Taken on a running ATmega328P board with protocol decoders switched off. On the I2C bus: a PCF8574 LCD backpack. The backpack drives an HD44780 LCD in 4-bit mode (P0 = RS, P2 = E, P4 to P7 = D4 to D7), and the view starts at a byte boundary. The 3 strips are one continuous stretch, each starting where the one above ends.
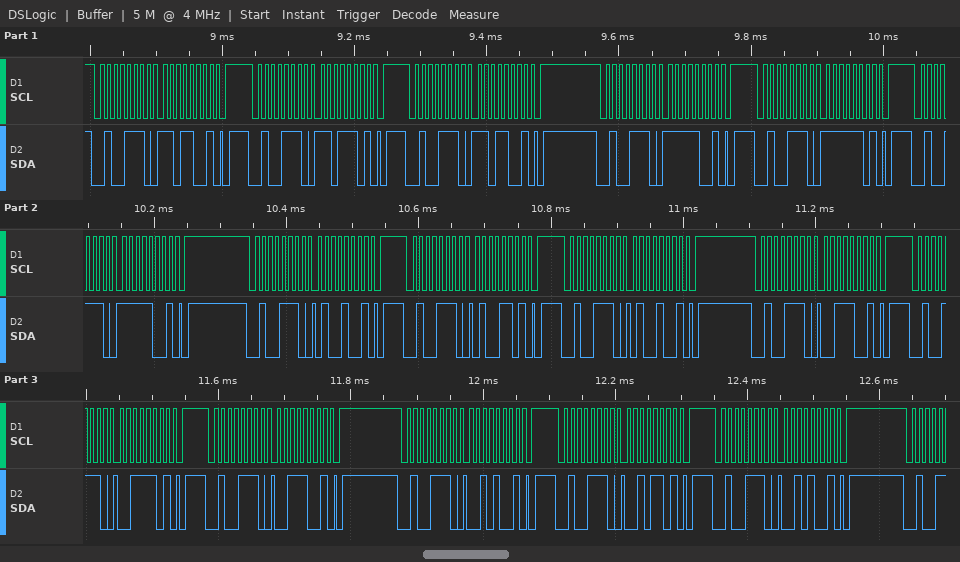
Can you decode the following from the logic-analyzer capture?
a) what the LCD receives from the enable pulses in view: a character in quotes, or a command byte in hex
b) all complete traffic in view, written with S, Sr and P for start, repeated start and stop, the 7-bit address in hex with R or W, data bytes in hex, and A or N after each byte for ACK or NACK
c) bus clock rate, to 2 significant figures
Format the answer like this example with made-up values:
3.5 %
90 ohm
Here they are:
data 0xDF 'C'
S 27W A D9 A P S 27W A DD A P S 27W A D9 A P S 27W A F9 A P S 27W A FD A P S 27W A F9 A P S 27W A 49 A P S 27W A 4D A P S 27W A 49 A P S 27W A 39 A P S 27W A 3D A P S 27W A 39 A P S 27W A 29 A P S 27W A 2D A P S 27W A 29 A P
100 kHz
